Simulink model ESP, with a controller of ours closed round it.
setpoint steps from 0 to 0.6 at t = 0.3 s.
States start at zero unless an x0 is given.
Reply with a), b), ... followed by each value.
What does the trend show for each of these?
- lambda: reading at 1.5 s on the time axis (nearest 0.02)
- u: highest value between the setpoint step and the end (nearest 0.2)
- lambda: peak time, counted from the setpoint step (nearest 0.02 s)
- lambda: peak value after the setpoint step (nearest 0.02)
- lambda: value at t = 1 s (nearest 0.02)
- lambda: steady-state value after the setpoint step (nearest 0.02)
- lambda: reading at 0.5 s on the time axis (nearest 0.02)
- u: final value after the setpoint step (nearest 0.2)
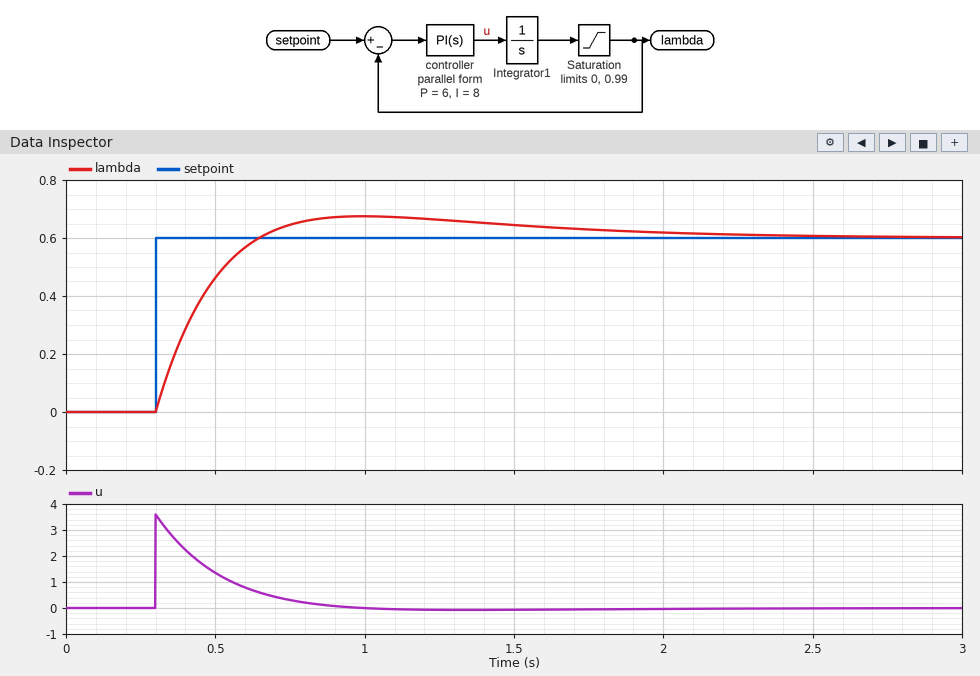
a) 0.64
b) 3.6
c) 0.70 s
d) 0.68
e) 0.68
f) 0.60
g) 0.46
h) 0.0
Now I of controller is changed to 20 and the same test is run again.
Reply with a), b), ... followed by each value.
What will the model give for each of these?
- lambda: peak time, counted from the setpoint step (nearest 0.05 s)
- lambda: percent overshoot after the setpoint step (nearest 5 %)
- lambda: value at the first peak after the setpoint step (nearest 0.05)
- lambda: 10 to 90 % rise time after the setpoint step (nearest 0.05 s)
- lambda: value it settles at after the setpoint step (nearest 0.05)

a) 0.50 s
b) 20 %
c) 0.75
d) 0.20 s
e) 0.60
